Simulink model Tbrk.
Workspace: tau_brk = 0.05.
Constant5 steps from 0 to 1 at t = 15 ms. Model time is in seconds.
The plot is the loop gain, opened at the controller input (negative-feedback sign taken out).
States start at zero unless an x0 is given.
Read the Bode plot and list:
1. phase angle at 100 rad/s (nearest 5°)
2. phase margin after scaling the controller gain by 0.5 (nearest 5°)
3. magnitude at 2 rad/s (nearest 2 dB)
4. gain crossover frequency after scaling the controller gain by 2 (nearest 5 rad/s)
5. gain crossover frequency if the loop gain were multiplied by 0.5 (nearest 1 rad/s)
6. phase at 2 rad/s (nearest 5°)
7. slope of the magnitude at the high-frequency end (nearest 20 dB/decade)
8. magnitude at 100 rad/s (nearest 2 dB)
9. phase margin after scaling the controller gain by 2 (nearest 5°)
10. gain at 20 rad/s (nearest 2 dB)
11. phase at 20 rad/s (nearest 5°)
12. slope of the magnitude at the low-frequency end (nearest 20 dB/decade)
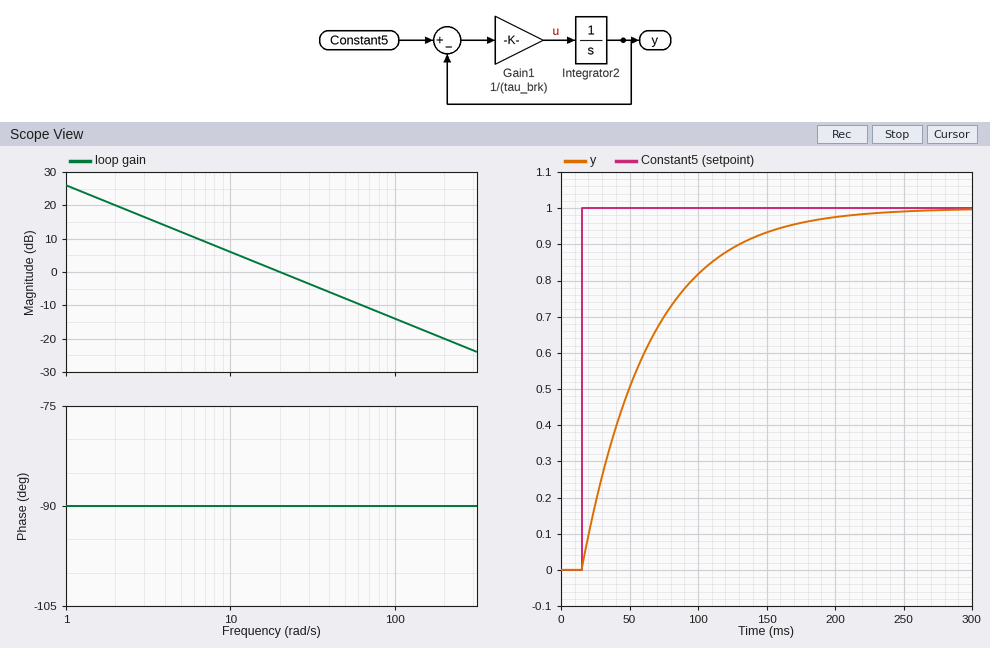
-90°
90°
20 dB
40 rad/s
10 rad/s
-90°
-20 dB/decade
-14 dB
90°
0 dB
-90°
-20 dB/decade
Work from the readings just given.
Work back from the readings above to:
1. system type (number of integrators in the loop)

1
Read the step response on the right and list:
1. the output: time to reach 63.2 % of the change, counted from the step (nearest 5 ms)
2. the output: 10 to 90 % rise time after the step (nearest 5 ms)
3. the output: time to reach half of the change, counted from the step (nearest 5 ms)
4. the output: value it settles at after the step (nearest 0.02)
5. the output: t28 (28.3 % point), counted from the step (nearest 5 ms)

50 ms
110 ms
35 ms
1.00
15 ms
